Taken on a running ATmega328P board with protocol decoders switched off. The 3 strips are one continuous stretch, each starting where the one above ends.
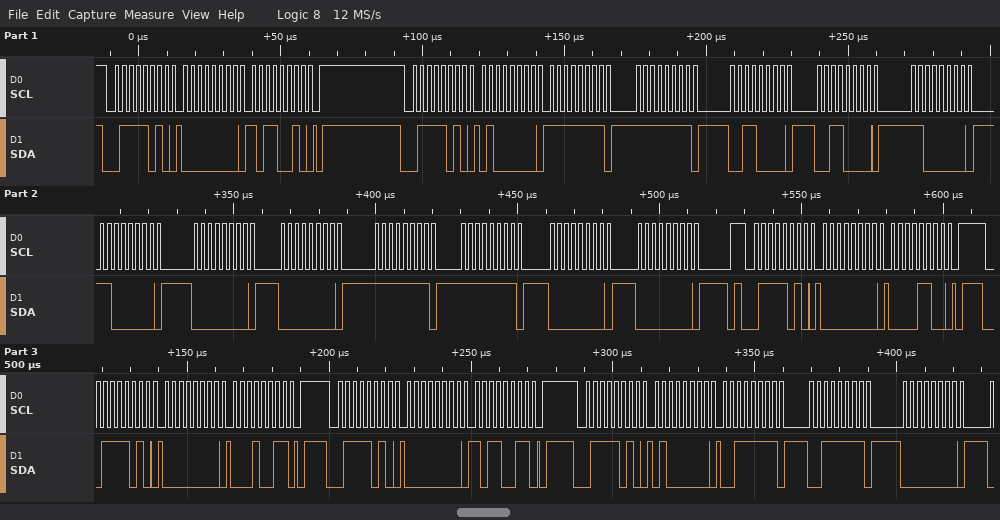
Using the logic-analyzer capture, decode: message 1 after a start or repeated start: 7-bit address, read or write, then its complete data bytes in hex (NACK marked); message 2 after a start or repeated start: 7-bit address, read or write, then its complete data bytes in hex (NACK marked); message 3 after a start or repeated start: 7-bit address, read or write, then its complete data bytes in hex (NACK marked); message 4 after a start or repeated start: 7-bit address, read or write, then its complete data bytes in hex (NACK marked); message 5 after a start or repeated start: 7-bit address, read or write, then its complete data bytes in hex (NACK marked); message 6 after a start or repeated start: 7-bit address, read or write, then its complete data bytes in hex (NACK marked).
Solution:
0x3D write: 00 B2
0x3D write: 40 FF FF 30 30 C0 C0 00 00 FF FF 00 00
0x3D write: 00 0C
0x3D write: 00 13
0x3D write: 00 B3
0x3D write: 40 3F 3F 00
